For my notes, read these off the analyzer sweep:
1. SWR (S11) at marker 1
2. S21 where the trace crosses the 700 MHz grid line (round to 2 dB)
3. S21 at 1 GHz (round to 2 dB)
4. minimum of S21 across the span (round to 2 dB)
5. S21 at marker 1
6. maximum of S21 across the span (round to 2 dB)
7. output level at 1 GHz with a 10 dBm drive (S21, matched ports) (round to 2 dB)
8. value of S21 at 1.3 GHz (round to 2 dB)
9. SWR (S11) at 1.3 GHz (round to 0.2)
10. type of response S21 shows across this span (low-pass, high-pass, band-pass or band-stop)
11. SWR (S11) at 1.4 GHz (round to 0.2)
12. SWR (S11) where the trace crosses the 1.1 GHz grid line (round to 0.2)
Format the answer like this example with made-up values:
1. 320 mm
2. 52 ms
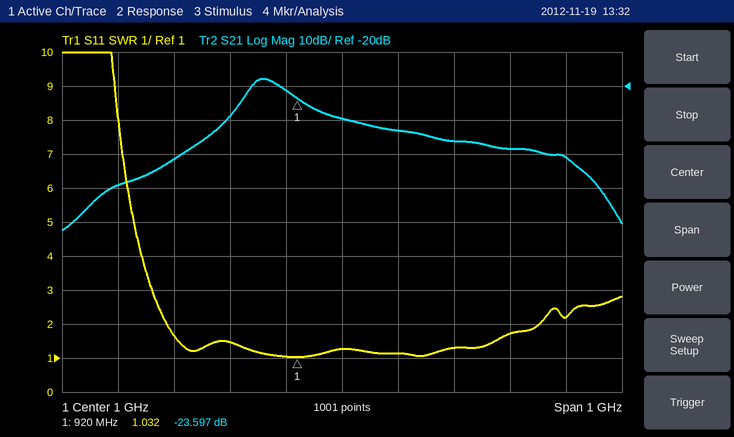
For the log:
1. 1.032
2. -42 dB
3. -30 dB
4. -62 dB
5. -23.597 dB
6. -18 dB
7. -20 dBm
8. -38 dB
9. 1.8
10. band-pass
11. 2.2
12. 1.2
